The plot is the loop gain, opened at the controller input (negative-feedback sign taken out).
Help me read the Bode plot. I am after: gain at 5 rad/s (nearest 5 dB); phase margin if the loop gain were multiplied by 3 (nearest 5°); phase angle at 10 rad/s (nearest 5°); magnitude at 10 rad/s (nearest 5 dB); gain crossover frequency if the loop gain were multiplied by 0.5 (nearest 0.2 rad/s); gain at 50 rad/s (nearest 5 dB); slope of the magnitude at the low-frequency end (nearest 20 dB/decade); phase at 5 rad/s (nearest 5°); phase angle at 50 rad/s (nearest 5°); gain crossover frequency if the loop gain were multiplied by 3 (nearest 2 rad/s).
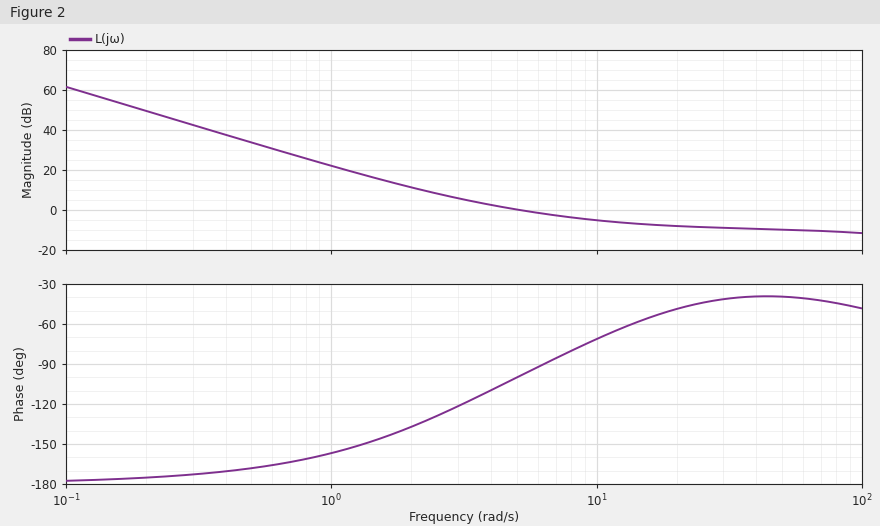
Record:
0 dB
140°
-70°
-5 dB
3.0 rad/s
-10 dB
-40 dB/decade
-100°
-40°
44 rad/s
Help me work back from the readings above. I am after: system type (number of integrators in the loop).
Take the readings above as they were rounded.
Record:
2
